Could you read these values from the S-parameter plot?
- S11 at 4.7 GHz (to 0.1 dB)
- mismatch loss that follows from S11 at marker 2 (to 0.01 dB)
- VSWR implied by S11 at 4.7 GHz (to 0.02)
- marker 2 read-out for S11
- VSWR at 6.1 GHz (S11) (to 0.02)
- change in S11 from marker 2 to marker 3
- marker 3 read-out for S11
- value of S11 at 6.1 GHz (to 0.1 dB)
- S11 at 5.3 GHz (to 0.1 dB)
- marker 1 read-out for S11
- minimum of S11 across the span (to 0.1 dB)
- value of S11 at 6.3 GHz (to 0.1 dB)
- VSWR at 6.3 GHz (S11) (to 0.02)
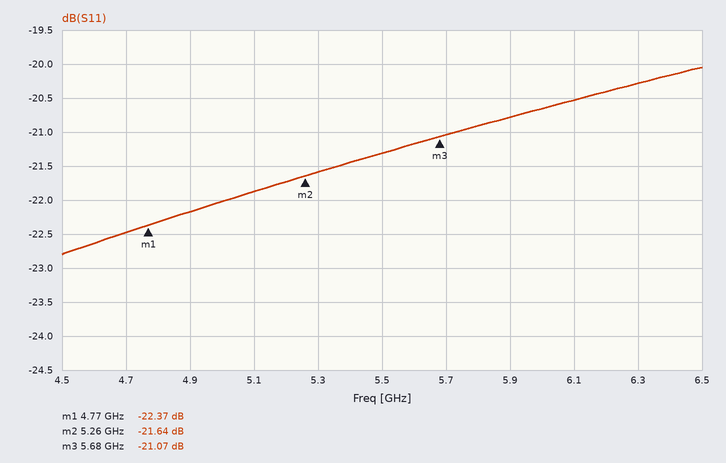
-22.5 dB
0.03 dB
1.16
-21.64 dB
1.20
0.57 dB
-21.07 dB
-20.5 dB
-21.6 dB
-22.37 dB
-22.8 dB
-20.3 dB
1.22
